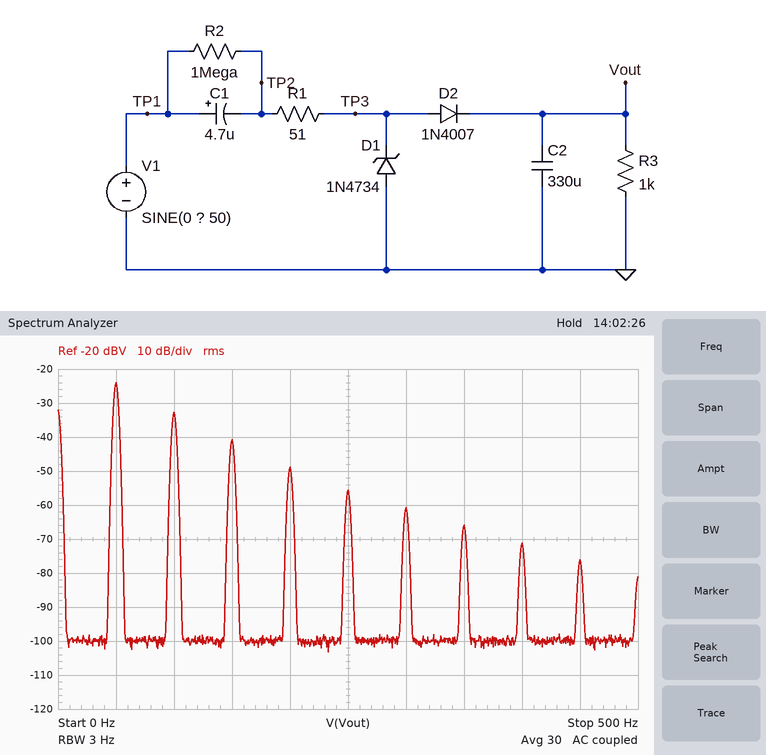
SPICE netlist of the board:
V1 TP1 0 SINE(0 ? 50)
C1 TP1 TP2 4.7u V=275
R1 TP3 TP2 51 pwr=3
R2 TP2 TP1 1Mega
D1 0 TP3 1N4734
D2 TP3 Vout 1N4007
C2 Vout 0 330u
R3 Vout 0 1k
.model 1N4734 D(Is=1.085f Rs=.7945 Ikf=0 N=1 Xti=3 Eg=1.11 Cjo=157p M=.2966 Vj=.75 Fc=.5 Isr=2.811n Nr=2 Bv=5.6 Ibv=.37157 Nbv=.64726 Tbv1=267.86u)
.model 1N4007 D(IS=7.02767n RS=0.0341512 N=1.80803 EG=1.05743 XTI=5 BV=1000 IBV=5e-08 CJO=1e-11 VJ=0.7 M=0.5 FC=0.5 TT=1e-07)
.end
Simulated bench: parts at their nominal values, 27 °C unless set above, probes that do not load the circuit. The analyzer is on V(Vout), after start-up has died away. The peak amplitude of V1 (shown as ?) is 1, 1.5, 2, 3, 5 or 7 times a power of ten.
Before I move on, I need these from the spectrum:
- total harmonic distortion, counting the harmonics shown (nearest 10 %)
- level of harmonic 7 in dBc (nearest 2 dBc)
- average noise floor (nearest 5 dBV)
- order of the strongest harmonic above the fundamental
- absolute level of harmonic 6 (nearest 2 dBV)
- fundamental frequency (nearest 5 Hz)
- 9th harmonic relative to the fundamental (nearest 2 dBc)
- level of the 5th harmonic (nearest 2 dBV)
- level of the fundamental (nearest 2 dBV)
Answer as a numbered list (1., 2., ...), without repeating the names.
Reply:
1. 40 %
2. -42 dBc
3. -100 dBV
4. 2
5. -60 dBV
6. 50 Hz
7. -52 dBc
8. -56 dBV
9. -24 dBV
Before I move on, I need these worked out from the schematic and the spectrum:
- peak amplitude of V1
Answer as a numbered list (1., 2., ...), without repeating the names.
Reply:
1. 300 V
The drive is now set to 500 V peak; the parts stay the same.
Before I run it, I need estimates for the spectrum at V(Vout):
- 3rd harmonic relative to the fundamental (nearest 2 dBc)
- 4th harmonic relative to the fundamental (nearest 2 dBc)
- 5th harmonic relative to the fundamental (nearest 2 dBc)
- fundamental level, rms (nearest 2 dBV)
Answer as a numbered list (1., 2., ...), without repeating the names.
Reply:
1. -14 dBc
2. -20 dBc
3. -28 dBc
4. -24 dBV
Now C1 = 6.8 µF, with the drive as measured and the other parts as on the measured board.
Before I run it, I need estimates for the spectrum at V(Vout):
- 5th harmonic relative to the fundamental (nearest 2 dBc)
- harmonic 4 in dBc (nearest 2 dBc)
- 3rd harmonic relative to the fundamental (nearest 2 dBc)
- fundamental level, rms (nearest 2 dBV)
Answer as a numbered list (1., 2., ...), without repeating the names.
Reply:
1. -28 dBc
2. -22 dBc
3. -14 dBc
4. -24 dBV
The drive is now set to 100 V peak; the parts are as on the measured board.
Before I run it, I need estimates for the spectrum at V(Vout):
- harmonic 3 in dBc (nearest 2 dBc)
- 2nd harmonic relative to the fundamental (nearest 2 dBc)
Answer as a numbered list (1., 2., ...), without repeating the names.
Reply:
1. -18 dBc
2. -10 dBc
